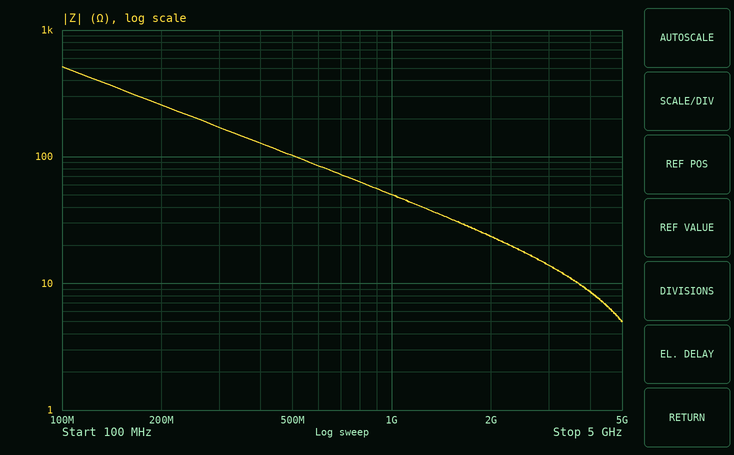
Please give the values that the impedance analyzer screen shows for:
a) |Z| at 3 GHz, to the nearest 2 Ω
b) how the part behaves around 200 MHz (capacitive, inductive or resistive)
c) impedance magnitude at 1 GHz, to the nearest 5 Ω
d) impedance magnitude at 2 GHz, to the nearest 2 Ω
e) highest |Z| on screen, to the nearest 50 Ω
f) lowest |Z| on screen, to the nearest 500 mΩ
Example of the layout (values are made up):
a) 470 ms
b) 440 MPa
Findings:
a) 14 Ω
b) capacitive
c) 50 Ω
d) 24 Ω
e) 500 Ω
f) 5.0 Ω
